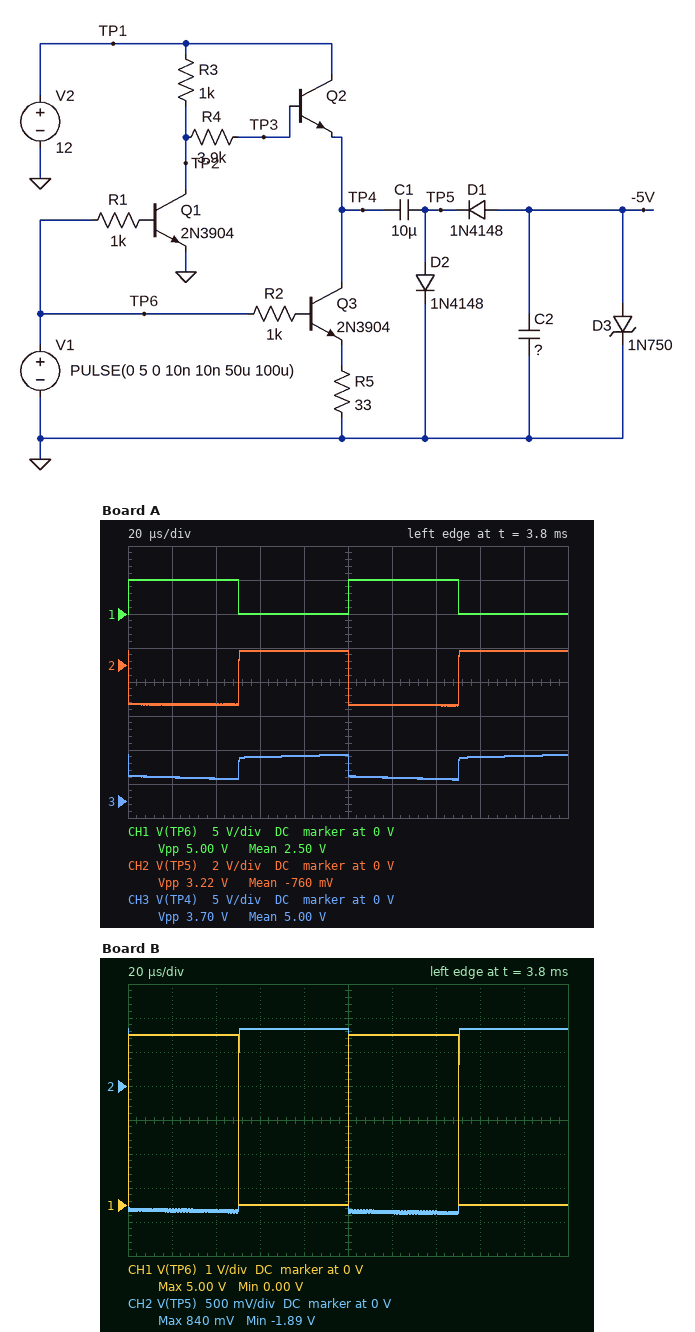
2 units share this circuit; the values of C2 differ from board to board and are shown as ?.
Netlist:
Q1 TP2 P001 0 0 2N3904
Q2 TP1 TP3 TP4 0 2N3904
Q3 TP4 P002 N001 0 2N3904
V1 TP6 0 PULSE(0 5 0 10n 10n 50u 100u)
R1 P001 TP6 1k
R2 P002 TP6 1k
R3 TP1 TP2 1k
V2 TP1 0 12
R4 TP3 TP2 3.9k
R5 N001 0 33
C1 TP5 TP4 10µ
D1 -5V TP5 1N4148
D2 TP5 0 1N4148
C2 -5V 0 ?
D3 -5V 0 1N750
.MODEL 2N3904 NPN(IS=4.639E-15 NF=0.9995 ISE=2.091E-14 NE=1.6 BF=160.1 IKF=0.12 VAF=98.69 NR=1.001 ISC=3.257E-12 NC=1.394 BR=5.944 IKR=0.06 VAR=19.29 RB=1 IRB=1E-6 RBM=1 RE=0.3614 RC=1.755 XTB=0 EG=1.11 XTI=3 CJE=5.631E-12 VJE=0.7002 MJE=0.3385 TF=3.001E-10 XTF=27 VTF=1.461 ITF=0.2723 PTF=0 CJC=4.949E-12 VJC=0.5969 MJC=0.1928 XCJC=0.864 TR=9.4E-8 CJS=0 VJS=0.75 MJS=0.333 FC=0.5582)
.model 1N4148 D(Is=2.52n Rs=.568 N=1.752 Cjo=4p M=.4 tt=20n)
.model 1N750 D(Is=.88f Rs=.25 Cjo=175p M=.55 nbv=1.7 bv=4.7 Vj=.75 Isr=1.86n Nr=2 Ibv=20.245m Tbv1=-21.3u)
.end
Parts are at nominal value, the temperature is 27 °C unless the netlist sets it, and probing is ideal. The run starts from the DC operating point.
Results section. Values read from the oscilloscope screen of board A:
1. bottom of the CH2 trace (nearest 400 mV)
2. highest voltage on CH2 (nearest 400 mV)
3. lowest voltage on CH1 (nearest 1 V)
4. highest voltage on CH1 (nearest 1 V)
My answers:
-2.4 V
800 mV
0 V
5 V
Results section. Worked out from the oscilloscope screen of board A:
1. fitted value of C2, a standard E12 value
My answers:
120 µF
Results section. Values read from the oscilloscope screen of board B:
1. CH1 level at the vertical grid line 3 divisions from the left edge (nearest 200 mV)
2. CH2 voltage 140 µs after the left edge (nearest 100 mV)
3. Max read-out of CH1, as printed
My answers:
0 V
-1.9 V
5.00 V
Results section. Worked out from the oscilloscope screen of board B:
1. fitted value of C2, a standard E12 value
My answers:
180 µF
